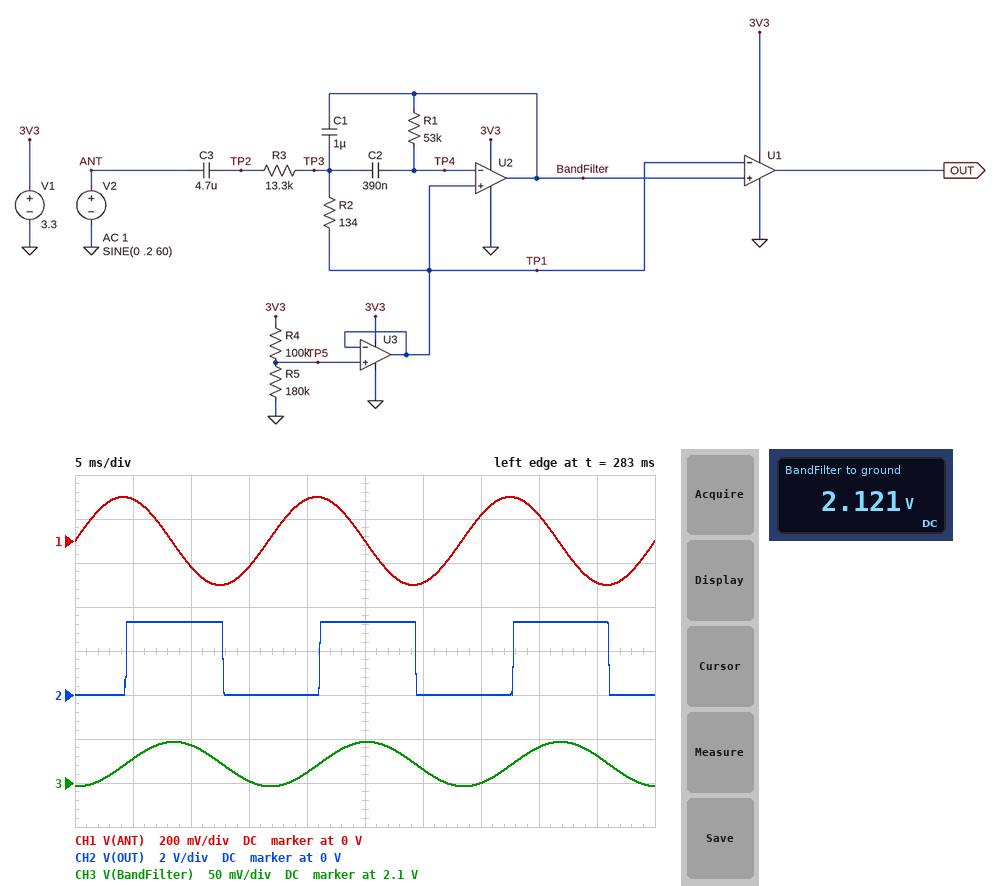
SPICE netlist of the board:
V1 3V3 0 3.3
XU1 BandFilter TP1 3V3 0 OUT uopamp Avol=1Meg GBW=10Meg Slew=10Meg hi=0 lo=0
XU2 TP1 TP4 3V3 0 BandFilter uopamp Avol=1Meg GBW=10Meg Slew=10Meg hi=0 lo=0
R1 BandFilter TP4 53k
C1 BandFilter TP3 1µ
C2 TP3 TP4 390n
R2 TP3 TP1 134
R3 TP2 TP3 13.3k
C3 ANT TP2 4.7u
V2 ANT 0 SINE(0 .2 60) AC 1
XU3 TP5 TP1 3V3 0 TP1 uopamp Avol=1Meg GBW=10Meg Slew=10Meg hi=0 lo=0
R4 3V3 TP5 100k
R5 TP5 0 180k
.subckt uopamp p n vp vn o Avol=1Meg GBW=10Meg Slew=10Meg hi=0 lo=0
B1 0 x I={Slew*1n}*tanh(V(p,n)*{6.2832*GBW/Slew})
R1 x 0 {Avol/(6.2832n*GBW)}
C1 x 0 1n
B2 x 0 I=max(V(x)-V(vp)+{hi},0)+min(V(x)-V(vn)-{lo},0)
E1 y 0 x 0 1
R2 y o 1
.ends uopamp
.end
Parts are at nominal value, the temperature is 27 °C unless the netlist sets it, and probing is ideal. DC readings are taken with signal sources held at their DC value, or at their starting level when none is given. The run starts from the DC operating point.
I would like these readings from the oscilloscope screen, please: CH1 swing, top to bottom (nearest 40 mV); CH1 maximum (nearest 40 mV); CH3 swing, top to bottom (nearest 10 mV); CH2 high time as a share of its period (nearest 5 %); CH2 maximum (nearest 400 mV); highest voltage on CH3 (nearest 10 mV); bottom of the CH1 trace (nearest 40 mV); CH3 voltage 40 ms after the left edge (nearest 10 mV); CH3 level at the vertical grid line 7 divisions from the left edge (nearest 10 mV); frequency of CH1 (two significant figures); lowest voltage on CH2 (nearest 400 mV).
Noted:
400 mV
200 mV
50 mV
50 %
3.2 V
2.15 V
-200 mV
2.14 V
2.10 V
60 Hz
0 V
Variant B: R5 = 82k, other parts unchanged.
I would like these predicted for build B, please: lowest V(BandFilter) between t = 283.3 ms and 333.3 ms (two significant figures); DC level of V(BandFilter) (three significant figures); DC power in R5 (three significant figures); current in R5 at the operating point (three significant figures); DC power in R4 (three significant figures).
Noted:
1.5 V
1.49 V
27.0 µW
18.1 µA
32.9 µW
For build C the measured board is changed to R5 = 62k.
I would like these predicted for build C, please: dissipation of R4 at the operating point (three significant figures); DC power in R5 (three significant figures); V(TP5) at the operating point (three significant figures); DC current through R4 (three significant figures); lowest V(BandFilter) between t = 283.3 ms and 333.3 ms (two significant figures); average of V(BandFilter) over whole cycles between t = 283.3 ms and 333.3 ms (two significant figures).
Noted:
41.5 µW
25.7 µW
1.26 V
20.4 µA
1.2 V
1.3 V
